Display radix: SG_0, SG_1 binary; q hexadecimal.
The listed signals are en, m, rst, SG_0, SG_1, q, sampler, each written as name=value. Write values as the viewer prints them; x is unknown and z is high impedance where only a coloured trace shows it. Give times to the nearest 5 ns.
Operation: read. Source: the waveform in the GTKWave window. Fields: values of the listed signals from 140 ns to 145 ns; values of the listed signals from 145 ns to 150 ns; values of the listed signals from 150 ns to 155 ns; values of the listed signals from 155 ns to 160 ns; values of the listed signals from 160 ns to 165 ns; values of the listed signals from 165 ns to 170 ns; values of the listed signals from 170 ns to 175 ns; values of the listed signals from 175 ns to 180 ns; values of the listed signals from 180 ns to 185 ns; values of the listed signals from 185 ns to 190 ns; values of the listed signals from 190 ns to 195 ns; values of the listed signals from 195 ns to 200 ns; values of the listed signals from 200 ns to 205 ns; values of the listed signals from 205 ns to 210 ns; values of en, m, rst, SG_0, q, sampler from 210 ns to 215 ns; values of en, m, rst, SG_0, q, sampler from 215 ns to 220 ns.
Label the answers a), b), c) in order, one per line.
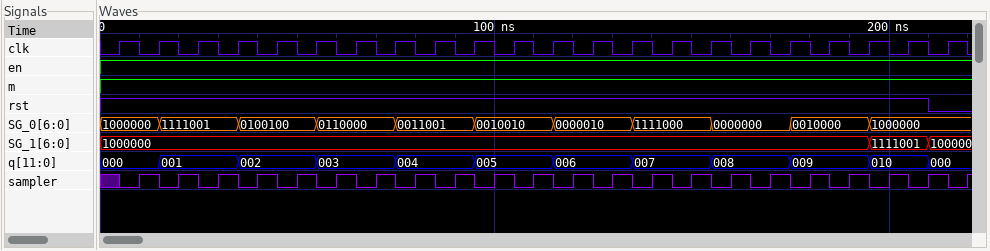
a) en=1, m=1, rst=1, SG_0=1111000, SG_1=1000000, q=007, sampler=1
b) en=1, m=1, rst=1, SG_0=1111000, SG_1=1000000, q=007, sampler=0
c) en=1, m=1, rst=1, SG_0=1111000, SG_1=1000000, q=007, sampler=1
d) en=1, m=1, rst=1, SG_0=0000000, SG_1=1000000, q=008, sampler=0
e) en=1, m=1, rst=1, SG_0=0000000, SG_1=1000000, q=008, sampler=1
f) en=1, m=1, rst=1, SG_0=0000000, SG_1=1000000, q=008, sampler=0
g) en=1, m=1, rst=1, SG_0=0000000, SG_1=1000000, q=008, sampler=1
h) en=1, m=1, rst=1, SG_0=0010000, SG_1=1000000, q=009, sampler=0
i) en=1, m=1, rst=1, SG_0=0010000, SG_1=1000000, q=009, sampler=1
j) en=1, m=1, rst=1, SG_0=0010000, SG_1=1000000, q=009, sampler=0
k) en=1, m=1, rst=1, SG_0=0010000, SG_1=1000000, q=009, sampler=1
l) en=1, m=1, rst=1, SG_0=1000000, SG_1=1111001, q=010, sampler=0
m) en=1, m=1, rst=1, SG_0=1000000, SG_1=1111001, q=010, sampler=1
n) en=1, m=1, rst=1, SG_0=1000000, SG_1=1111001, q=010, sampler=0
o) en=1, m=1, rst=0, SG_0=1000000, q=000, sampler=1
p) en=1, m=1, rst=0, SG_0=1000000, q=000, sampler=0
